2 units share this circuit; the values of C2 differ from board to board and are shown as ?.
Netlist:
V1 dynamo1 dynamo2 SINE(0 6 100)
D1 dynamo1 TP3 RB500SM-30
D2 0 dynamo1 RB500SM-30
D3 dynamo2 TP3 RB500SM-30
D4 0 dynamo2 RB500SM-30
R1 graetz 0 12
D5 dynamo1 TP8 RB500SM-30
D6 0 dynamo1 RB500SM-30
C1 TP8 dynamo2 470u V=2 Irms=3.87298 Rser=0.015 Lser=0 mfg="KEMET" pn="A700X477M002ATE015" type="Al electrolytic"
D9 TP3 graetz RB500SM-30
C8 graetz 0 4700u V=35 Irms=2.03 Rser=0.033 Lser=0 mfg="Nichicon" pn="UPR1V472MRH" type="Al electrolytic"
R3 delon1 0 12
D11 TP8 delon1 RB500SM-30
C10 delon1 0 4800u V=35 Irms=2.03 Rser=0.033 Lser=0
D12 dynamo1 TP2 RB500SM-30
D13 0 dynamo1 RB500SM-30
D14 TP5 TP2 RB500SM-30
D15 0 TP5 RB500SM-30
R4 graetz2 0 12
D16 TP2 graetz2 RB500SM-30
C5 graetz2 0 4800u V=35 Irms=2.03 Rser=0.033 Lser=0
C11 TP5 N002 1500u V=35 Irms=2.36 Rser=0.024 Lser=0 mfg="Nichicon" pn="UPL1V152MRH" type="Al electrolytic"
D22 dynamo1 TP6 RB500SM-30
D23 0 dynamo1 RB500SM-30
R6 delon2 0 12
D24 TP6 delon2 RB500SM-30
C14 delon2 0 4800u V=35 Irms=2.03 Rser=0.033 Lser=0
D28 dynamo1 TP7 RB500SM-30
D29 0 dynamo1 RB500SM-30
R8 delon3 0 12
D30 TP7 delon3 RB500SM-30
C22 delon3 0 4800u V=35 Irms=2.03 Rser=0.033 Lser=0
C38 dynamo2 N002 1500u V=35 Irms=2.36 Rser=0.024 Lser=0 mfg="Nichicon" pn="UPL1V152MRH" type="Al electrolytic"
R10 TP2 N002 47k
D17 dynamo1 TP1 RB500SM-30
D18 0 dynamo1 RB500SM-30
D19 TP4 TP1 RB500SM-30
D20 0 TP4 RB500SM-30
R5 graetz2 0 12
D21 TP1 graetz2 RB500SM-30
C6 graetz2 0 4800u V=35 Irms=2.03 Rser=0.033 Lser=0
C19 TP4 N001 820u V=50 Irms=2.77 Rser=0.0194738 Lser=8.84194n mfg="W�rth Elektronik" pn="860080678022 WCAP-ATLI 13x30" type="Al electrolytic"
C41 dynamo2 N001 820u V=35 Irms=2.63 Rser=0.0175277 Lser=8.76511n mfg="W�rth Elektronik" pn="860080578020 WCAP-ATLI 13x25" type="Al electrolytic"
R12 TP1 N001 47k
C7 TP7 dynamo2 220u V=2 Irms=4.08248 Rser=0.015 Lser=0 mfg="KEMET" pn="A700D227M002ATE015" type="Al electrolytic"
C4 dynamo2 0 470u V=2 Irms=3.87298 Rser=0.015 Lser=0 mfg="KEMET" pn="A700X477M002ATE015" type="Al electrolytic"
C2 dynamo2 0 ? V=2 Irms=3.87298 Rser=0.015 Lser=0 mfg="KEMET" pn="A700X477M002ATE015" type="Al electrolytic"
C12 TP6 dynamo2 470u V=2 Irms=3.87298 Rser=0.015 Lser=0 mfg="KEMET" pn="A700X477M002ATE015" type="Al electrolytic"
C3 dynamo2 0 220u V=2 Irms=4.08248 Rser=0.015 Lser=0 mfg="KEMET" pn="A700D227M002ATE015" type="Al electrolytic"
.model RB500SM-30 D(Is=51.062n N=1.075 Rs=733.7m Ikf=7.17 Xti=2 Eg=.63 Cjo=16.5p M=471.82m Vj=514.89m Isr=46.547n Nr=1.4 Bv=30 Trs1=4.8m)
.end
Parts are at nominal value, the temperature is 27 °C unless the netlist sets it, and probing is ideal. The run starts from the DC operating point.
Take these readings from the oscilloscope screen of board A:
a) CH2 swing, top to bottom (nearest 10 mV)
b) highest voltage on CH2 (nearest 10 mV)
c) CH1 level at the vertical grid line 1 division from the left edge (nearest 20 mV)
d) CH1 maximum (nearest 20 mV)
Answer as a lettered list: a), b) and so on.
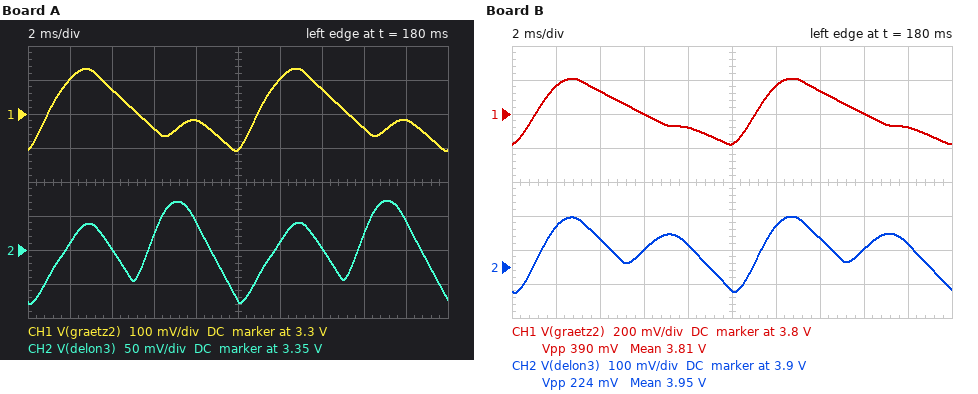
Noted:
a) 150 mV
b) 3.42 V
c) 3.40 V
d) 3.44 V
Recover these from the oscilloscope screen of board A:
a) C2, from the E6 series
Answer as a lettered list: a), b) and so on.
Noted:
a) 330 µF
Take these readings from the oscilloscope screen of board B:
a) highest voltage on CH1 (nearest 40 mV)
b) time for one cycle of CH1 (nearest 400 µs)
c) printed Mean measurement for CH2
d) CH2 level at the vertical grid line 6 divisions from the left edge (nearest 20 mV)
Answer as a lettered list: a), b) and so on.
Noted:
a) 4.00 V
b) 10.0 ms
c) 3.95 V
d) 4.02 V
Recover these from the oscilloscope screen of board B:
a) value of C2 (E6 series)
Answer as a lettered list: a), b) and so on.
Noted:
a) 1.5 mF
